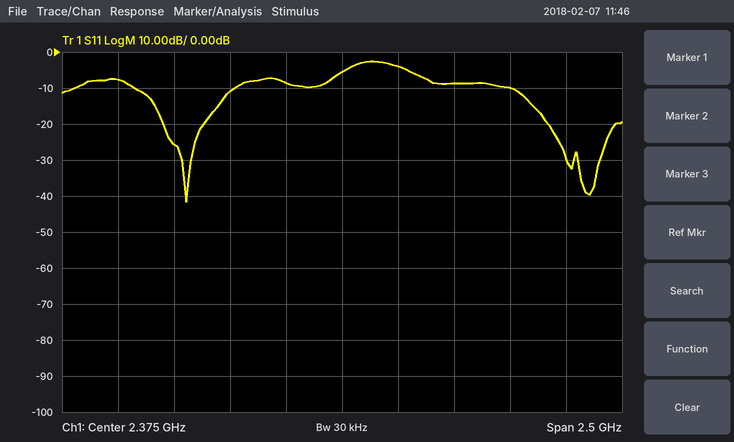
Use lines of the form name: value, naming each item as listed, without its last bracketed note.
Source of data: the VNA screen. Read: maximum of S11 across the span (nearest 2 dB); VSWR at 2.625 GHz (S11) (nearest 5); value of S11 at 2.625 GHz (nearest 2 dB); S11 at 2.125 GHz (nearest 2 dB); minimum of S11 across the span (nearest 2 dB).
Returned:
maximum of S11 across the span: -2 dB
VSWR at 2.625 GHz (S11): 5
value of S11 at 2.625 GHz: -4 dB
S11 at 2.125 GHz: -8 dB
minimum of S11 across the span: -42 dB
